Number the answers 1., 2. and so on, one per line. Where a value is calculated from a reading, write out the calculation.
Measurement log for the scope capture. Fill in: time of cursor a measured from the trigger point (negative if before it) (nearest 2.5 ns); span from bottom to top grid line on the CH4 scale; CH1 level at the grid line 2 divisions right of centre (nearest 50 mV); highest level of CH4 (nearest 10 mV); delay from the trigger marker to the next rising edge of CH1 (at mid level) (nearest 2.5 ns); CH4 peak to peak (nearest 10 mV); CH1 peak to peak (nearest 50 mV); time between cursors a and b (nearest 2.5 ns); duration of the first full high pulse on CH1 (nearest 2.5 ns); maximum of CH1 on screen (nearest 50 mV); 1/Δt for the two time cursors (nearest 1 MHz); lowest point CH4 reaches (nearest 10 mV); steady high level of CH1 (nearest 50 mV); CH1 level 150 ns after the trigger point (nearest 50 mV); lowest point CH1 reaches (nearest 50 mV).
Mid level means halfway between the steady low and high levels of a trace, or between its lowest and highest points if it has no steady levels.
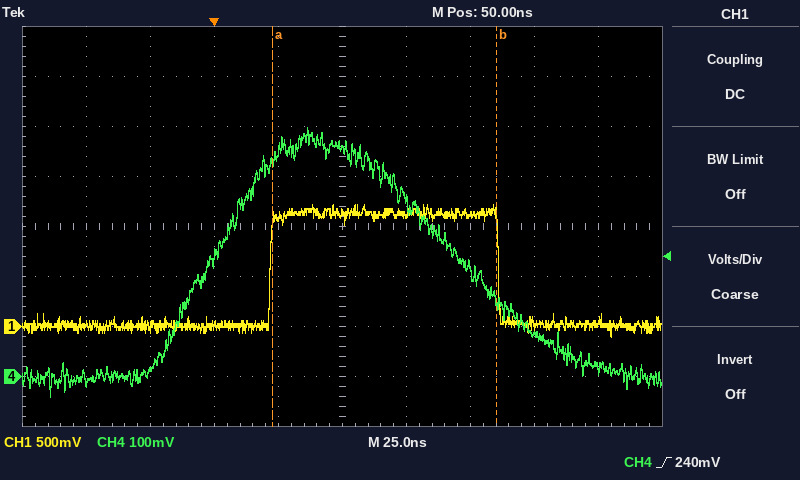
1. +22.5 ns
2. 800 mV
3. 1.10 V
4. 500 mV
5. 22.5 ns
6. 500 mV − (-40 mV) = 540 mV
7. 1.20 V − (-100 mV) = 1.30 V
8. 87.5 ns
9. 90.0 ns
10. 1.20 V
11. 1 / 87.5 ns ≈ 11 MHz
12. -40 mV
13. 1.15 V
14. 50 mV
15. -100 mV
